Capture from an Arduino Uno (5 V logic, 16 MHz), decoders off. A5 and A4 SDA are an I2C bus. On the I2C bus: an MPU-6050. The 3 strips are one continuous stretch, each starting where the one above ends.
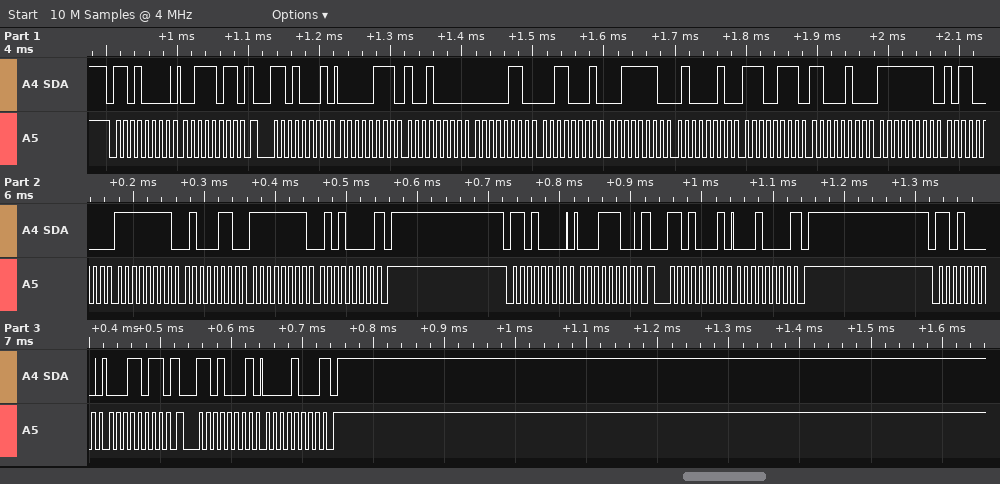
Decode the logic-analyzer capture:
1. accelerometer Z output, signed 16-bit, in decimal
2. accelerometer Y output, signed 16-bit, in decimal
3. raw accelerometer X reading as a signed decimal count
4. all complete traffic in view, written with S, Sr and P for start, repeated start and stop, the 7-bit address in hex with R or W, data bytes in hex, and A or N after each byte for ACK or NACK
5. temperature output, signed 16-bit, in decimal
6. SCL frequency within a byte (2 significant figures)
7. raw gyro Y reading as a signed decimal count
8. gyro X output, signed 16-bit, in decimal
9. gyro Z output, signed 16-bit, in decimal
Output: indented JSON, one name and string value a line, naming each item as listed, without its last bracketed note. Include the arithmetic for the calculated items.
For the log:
{
  "accelerometer Z output, signed 16-bit, in decimal": "0x3E42 = 15938",
  "accelerometer Y output, signed 16-bit, in decimal": "0x0631 = 1585",
  "raw accelerometer X reading as a signed decimal count": "0x0790 = 1936",
  "all complete traffic in view, written with S, Sr and P for start, repeated start and stop, the 7-bit address in hex with R or W, data bytes in hex, and A or N after each byte for ACK or NACK": "S 68W A 3B A Sr 68R A 07 A 90 A 06 A 31 A 3E A 42 A E7 A C4 A FF A B0 A FF A 46 A FF A 50 N P S 68W A 1C A Sr 68R A 10 N P S 68W A 1B A Sr 68R A 08 N P",
  "temperature output, signed 16-bit, in decimal": "0xE7C4 = -6204",
  "SCL frequency within a byte": "100 kHz",
  "raw gyro Y reading as a signed decimal count": "0xFF46 = -186",
  "gyro X output, signed 16-bit, in decimal": "0xFFB0 = -80",
  "gyro Z output, signed 16-bit, in decimal": "0xFF50 = -176"
}
